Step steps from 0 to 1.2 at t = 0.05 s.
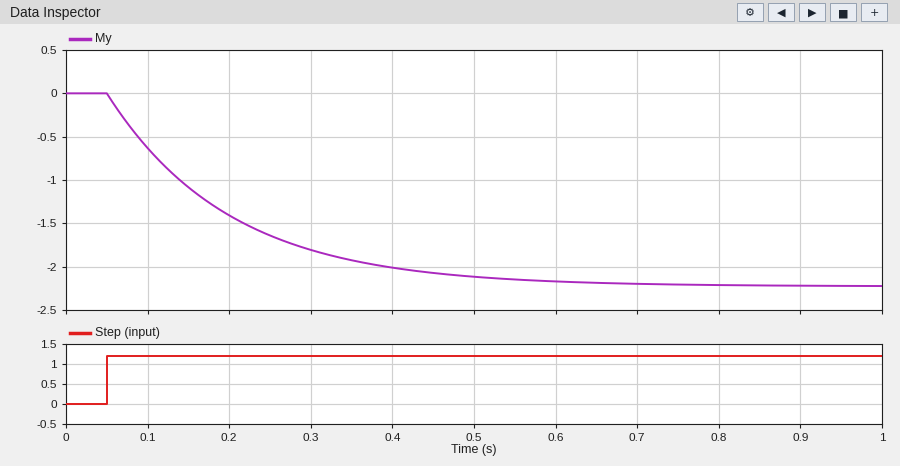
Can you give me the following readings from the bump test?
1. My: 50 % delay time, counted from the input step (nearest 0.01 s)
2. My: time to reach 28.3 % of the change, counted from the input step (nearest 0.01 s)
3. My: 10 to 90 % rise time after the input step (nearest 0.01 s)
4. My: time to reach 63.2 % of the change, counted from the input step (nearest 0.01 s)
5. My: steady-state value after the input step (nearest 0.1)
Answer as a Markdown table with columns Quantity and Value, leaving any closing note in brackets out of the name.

| Quantity | Value |
|---|---|
| My: 50 % delay time, counted from the input step | 0.10 s |
| My: time to reach 28.3 % of the change, counted from the input step | 0.05 s |
| My: 10 to 90 % rise time after the input step | 0.33 s |
| My: time to reach 63.2 % of the change, counted from the input step | 0.15 s |
| My: steady-state value after the input step | -2.2 |
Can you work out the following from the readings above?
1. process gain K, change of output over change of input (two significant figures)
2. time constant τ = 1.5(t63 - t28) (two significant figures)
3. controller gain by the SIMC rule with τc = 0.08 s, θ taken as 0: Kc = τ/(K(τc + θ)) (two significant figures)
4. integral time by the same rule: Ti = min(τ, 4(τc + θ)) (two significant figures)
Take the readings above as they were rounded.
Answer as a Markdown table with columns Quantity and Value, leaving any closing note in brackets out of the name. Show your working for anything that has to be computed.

| Quantity | Value |
|---|---|
| process gain K, change of output over change of input | (-2.2 - 0) / 1.2 = -1.8 |
| time constant τ = 1.5(t63 - t28) | 1.5 × (0.15 - 0.05) = 0.15 s |
| controller gain by the SIMC rule with τc = 0.08 s, θ taken as 0: Kc = τ/(K(τc + θ)) | 0.15 / (-1.8 × (0.08 + 0)) = -1.0 |
| integral time by the same rule: Ti = min(τ, 4(τc + θ)) | min(0.15, 4 × (0.08 + 0)) = 0.15 s |
